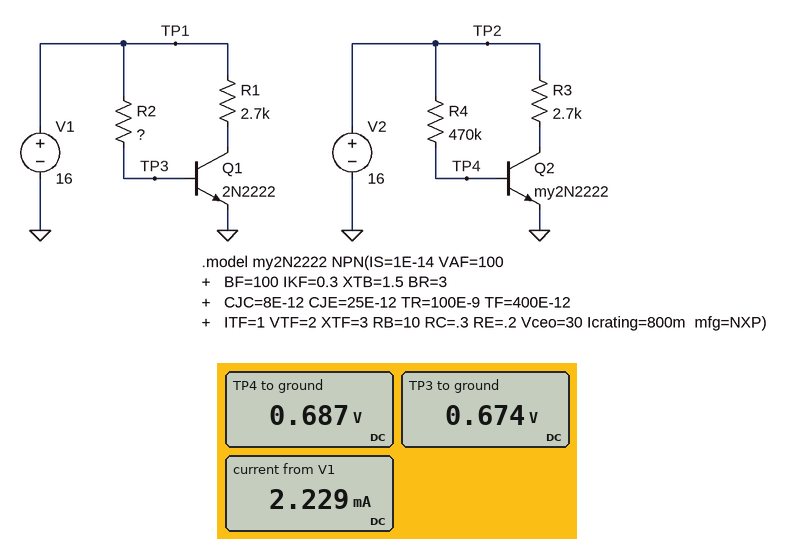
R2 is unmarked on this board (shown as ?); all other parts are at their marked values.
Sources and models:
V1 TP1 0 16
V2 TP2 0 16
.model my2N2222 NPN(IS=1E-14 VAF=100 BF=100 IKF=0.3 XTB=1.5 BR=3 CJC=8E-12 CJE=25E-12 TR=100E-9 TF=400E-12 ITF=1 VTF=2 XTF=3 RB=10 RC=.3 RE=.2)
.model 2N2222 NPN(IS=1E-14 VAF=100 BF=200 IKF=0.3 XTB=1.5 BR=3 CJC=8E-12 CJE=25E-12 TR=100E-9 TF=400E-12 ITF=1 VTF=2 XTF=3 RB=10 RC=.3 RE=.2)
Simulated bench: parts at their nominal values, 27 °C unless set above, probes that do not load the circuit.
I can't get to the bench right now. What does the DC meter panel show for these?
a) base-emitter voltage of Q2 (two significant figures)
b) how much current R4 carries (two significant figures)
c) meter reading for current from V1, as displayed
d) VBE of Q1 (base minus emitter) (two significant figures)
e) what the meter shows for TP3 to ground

690 mV
33 µA
2.229 mA
670 mV
0.674 V
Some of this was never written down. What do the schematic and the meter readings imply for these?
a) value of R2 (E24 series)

1.5 MΩ
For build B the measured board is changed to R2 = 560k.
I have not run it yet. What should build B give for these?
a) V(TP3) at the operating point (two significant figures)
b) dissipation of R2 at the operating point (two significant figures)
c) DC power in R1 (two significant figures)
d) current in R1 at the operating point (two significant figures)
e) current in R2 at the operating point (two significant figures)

700 mV
420 µW
79 mW
5.4 mA
27 µA
